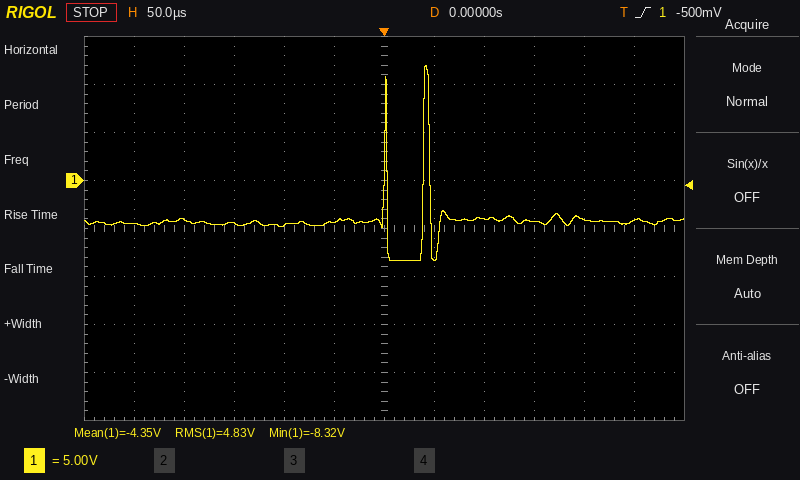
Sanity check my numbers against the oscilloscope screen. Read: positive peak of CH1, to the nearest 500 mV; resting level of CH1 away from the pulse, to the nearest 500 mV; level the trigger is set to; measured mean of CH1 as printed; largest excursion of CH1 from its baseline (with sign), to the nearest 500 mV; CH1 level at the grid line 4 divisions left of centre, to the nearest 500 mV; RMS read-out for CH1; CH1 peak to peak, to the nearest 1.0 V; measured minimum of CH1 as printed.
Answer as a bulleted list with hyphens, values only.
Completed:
- 12.0 V
- -4.5 V
- -500 mV
- -4.35 V
- +16.5 V
- -4.0 V
- 4.83 V
- 20.0 V
- -8.32 V
